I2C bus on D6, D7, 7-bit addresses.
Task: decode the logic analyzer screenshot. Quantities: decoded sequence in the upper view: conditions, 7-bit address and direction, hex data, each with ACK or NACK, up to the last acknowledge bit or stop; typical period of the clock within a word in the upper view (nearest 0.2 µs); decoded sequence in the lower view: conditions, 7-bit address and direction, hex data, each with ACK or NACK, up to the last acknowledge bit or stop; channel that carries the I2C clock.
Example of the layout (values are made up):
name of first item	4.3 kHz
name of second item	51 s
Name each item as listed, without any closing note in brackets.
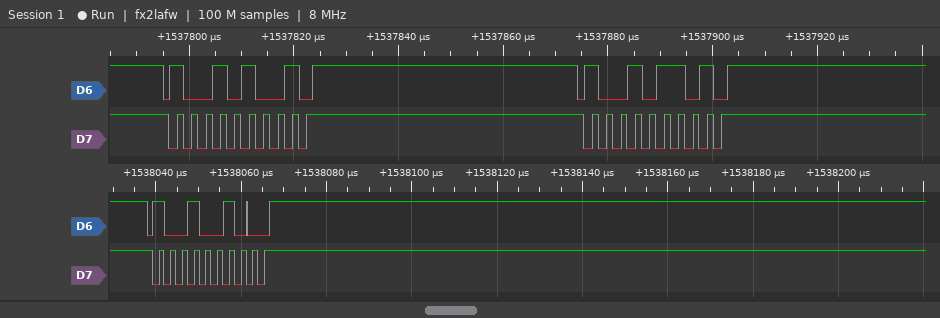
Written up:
decoded sequence in the upper view: conditions, 7-bit address and direction, hex data, each with ACK or NACK, up to the last acknowledge bit or stop	start, address 4A write NACK, stop, start, address 4B write NACK, stop
typical period of the clock within a word in the upper view	2.8 µs
decoded sequence in the lower view: conditions, 7-bit address and direction, hex data, each with ACK or NACK, up to the last acknowledge bit or stop	start, address 49 write ACK, stop
channel that carries the I2C clock	D7
